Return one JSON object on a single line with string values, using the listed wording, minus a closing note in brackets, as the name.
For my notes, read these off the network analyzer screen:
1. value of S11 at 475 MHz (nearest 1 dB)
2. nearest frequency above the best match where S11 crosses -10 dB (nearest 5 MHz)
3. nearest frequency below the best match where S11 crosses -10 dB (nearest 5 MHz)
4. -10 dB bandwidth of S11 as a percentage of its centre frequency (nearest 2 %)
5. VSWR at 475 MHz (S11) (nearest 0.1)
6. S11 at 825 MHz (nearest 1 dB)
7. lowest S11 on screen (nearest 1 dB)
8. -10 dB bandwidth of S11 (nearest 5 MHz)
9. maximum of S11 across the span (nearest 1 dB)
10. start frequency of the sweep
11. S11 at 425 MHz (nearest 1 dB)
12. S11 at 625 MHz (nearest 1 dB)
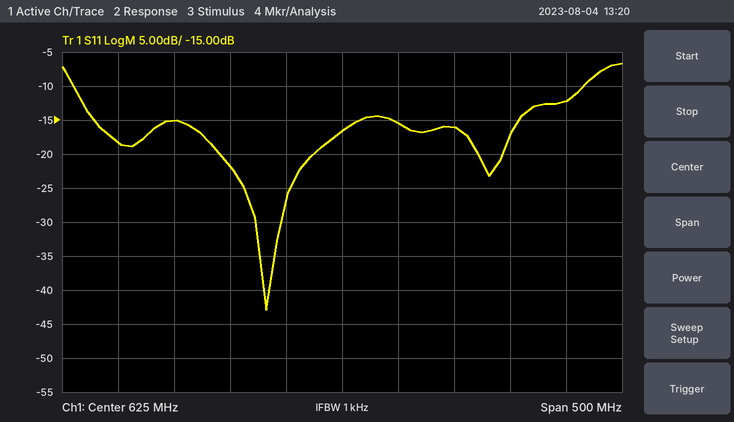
{"value of S11 at 475 MHz": "-15 dB", "nearest frequency above the best match where S11 crosses -10 dB": "840 MHz", "nearest frequency below the best match where S11 crosses -10 dB": "385 MHz", "-10 dB bandwidth of S11 as a percentage of its centre frequency": "74 %", "VSWR at 475 MHz (S11)": "1.4", "S11 at 825 MHz": "-12 dB", "lowest S11 on screen": "-43 dB", "-10 dB bandwidth of S11": "455 MHz", "maximum of S11 across the span": "-7 dB", "start frequency of the sweep": "375 MHz", "S11 at 425 MHz": "-18 dB", "S11 at 625 MHz": "-17 dB"}
